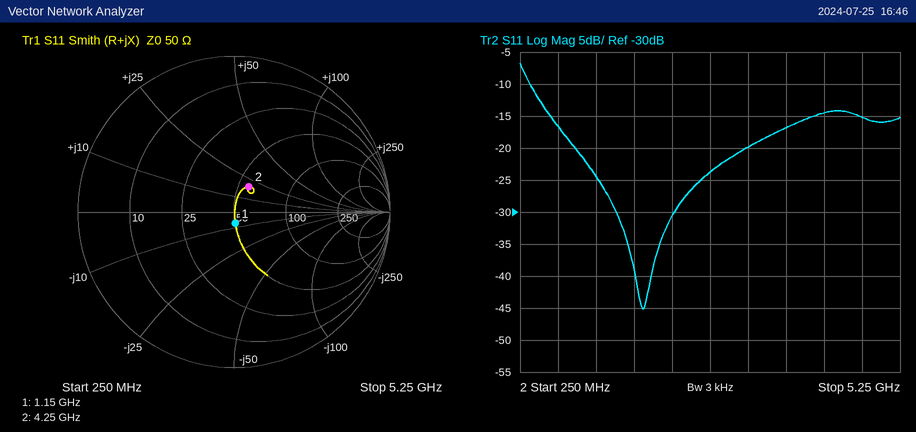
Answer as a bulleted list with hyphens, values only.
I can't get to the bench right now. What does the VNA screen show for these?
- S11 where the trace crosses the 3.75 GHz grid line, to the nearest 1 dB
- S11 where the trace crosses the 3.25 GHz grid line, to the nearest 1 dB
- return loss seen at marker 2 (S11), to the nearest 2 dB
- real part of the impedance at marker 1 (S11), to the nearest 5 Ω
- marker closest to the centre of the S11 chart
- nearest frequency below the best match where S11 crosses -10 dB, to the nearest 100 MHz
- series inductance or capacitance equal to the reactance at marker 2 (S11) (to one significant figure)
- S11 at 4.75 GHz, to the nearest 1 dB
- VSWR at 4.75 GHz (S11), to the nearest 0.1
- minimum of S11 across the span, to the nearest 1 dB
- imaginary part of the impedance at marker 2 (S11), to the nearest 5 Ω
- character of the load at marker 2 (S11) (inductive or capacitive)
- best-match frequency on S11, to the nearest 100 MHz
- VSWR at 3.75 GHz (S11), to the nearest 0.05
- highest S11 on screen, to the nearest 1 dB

- -17 dB
- -20 dB
- 14 dB
- 50 Ω
- marker 1
- 400 MHz
- 700 pH
- -15 dB
- 1.4
- -45 dB
- +20 Ω
- inductive
- 1.9 GHz
- 1.35
- -7 dB
